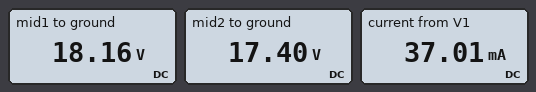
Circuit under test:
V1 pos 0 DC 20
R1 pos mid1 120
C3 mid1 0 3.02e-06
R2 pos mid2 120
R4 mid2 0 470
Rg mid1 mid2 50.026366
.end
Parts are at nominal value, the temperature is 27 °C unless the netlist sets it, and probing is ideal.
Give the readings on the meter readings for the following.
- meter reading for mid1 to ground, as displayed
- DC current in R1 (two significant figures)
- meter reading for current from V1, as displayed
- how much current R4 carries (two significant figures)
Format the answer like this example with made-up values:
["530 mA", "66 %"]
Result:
["18.16 V", "15 mA", "37.01 mA", "37 mA"]
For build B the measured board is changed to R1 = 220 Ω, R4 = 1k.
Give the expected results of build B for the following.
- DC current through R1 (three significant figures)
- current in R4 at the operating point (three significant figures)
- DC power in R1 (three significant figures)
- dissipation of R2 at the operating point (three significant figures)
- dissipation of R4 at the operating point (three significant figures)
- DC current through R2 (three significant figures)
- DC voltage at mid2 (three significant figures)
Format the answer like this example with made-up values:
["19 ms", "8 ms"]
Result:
["5.68 mA", "18.5 mA", "7.10 mW", "19.6 mW", "341 mW", "12.8 mA", "18.5 V"]
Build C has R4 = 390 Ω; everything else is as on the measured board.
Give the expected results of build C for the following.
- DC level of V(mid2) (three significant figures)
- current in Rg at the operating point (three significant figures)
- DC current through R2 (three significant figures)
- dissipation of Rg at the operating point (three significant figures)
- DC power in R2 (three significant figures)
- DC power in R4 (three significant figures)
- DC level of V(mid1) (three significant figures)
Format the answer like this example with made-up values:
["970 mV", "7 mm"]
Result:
["16.9 V", "18.0 mA", "25.5 mA", "16.2 mW", "77.8 mW", "736 mW", "17.8 V"]
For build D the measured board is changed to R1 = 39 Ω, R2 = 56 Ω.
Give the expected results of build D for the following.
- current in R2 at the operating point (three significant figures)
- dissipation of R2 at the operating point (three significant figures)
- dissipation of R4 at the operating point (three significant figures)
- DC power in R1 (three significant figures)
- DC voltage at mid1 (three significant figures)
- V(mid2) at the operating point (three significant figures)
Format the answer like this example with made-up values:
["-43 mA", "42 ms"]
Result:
["24.3 mA", "33.2 mW", "739 mW", "9.14 mW", "19.4 V", "18.6 V"]
